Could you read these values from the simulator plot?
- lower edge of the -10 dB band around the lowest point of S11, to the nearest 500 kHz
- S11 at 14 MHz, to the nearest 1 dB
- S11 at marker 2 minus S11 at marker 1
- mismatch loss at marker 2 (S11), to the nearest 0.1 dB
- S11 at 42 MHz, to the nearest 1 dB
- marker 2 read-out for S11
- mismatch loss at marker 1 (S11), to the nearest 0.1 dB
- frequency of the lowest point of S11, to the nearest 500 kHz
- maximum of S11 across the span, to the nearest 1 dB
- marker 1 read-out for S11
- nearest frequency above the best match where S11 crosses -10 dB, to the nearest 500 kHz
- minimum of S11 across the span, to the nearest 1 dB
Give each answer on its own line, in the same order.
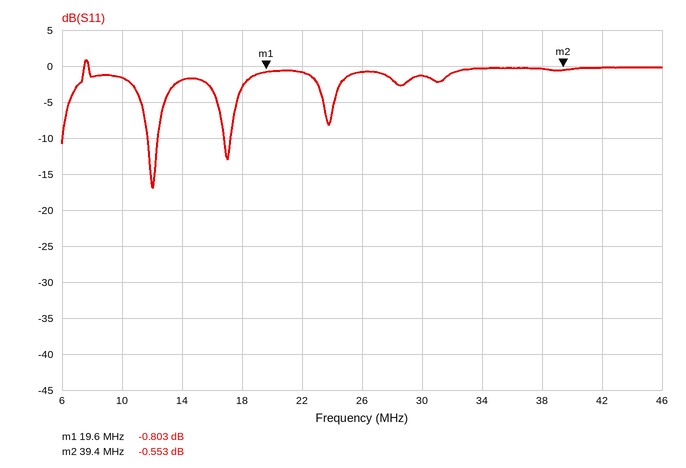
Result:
11.5 MHz
-2 dB
0.250 dB
9.2 dB
0 dB
-0.553 dB
7.7 dB
12.0 MHz
1 dB
-0.803 dB
12.5 MHz
-17 dB
